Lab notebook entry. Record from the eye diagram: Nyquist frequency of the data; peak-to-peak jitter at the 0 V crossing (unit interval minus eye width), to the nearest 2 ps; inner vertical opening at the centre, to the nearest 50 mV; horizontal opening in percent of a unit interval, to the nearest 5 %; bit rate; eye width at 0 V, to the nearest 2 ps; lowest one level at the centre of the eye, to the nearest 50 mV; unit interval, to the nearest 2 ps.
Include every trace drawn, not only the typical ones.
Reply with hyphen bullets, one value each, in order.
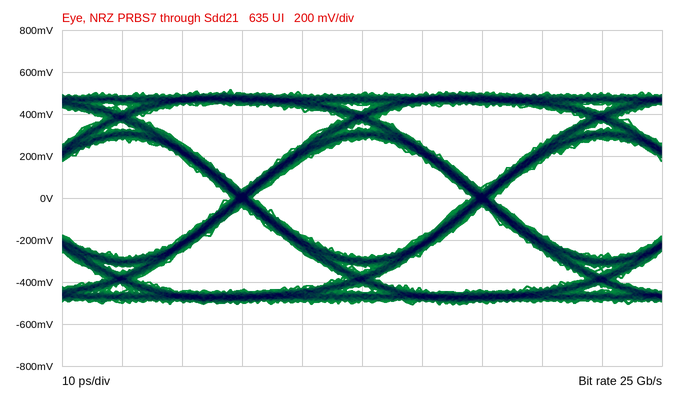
- 12.5 GHz
- 4 ps
- 550 mV
- 90 %
- 25 Gb/s
- 36 ps
- 300 mV
- 40 ps
